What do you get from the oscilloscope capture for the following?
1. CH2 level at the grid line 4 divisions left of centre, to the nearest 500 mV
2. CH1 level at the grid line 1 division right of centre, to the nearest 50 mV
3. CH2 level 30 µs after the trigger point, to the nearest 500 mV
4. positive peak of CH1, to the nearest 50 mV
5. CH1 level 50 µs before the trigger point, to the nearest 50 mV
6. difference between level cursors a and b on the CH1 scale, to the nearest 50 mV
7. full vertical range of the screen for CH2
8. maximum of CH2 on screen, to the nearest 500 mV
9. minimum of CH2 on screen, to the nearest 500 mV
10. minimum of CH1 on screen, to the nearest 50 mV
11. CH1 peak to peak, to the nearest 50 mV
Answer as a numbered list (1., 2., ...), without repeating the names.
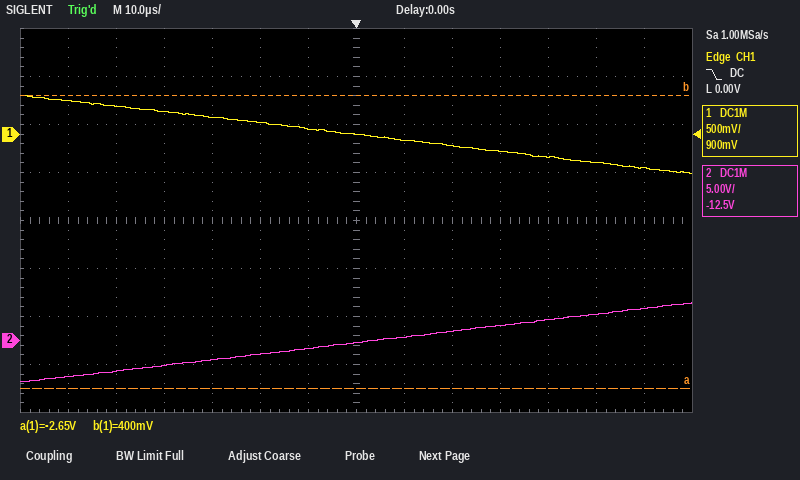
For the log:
1. -2.5 V
2. -50 mV
3. 1.5 V
4. 400 mV
5. 300 mV
6. 3.05 V
7. 40 V
8. 4.0 V
9. -4.5 V
10. -400 mV
11. 800 mV
